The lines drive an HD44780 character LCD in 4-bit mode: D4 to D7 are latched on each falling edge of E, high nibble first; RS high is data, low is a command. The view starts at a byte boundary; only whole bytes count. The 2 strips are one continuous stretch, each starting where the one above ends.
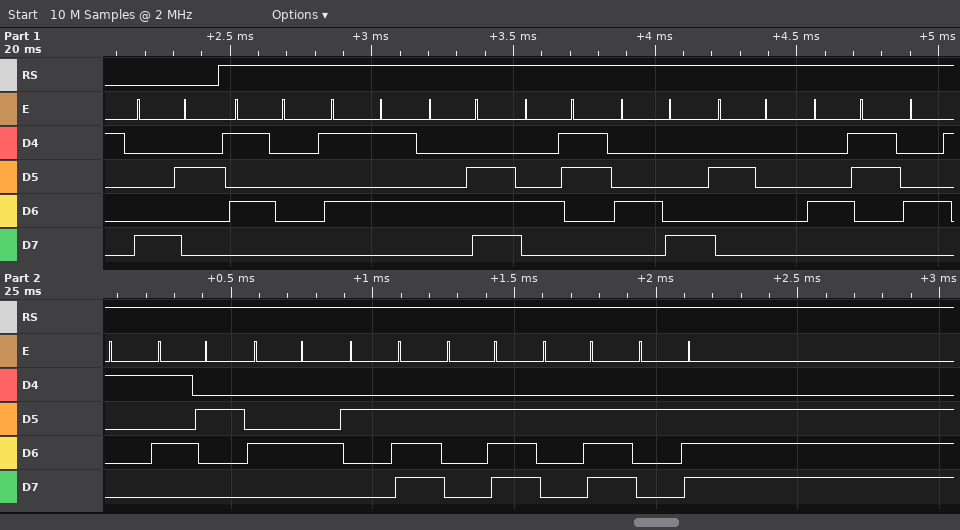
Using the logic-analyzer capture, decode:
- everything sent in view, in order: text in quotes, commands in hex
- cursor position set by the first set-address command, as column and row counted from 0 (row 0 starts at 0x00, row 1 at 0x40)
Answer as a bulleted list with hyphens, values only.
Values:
- 0x82 "PUNCH CARD...."
- column 2, row 0
